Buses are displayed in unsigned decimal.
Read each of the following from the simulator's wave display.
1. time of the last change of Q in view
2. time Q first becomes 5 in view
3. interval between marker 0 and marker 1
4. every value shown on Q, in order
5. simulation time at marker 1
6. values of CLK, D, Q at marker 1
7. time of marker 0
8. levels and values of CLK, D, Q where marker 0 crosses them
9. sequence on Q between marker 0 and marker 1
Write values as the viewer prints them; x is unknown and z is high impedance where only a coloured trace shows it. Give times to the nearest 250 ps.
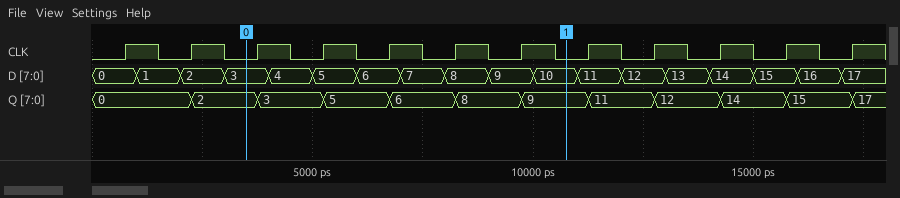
17250 ps
5250 ps
7250 ps
0, 2, 3, 5, 6, 8, 9, 11, 12, 14, 15, 17
10750 ps
CLK=0, D=10, Q=9
3500 ps
CLK=0, D=3, Q=2
2, 3, 5, 6, 8, 9
